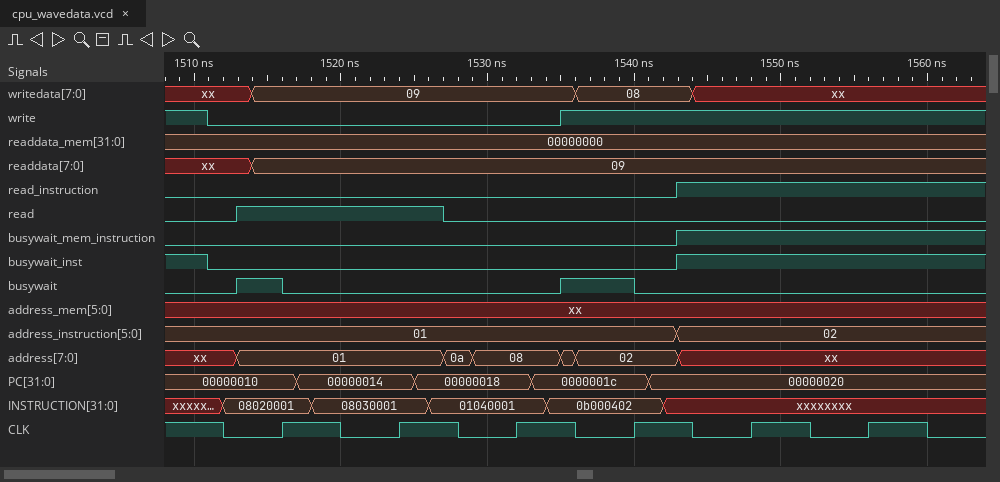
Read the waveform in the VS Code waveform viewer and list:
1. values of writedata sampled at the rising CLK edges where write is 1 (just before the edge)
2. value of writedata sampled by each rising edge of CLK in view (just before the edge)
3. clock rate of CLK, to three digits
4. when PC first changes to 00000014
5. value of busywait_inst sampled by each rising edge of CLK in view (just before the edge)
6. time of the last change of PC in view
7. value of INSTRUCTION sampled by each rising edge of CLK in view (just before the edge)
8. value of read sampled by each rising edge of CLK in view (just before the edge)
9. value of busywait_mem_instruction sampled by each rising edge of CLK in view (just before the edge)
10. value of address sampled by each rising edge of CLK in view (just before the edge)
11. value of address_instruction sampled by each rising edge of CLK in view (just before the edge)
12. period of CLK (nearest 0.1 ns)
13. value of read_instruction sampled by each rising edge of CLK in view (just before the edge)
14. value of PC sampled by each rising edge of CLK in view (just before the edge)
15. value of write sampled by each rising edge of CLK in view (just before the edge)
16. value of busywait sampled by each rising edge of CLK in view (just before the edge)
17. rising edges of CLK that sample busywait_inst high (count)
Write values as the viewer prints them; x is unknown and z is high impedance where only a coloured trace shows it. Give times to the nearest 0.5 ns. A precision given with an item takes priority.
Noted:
08, xx, xx
09, 09, 09, 08, xx, xx
125 MHz
1517 ns
0 0 0 0 1 1
1541 ns
08020001, 08030001, 01040001, 0b000402, xxxxxxxx, xxxxxxxx
1 1 0 0 0 0
0 0 0 0 1 1
01, 01, 08, 02, xx, xx
01, 01, 01, 01, 02, 02
8 ns
0 0 0 0 1 1
00000010, 00000014, 00000018, 0000001c, 00000020, 00000020
0 0 0 1 1 1
1 0 0 1 0 0
2
